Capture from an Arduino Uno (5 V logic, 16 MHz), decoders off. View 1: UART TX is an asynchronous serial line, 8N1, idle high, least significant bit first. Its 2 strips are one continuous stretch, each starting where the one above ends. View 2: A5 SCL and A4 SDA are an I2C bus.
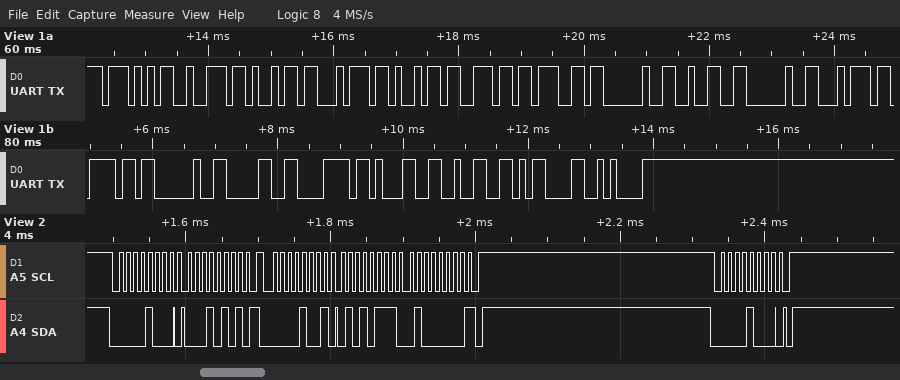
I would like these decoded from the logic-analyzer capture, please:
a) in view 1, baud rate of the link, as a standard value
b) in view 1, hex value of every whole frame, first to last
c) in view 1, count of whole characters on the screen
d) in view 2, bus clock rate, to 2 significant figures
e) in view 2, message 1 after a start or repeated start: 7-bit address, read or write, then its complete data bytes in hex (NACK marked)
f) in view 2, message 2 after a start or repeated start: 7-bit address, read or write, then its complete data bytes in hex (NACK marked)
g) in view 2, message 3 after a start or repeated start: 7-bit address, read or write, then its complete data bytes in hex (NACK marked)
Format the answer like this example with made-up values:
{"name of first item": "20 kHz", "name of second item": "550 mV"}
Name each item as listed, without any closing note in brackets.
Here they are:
{"in view 1, baud rate of the link, as a standard value": "9600 baud", "in view 1, hex value of every whole frame, first to last": "57 72 69 74 69 6E 67 20 32 20 74 6F 20 30 78 31 32 0D 0A", "in view 1, count of whole characters on the screen": "19", "in view 2, bus clock rate, to 2 significant figures": "100 kHz", "in view 2, message 1 after a start or repeated start: 7-bit address, read or write, then its complete data bytes in hex": "0x04 write: 15", "in view 2, message 2 after a start or repeated start: 7-bit address, read or write, then its complete data bytes in hex": "0x04 read: 57 40 NACK", "in view 2, message 3 after a start or repeated start: 7-bit address, read or write, then its complete data bytes in hex": "0x04 write"}
